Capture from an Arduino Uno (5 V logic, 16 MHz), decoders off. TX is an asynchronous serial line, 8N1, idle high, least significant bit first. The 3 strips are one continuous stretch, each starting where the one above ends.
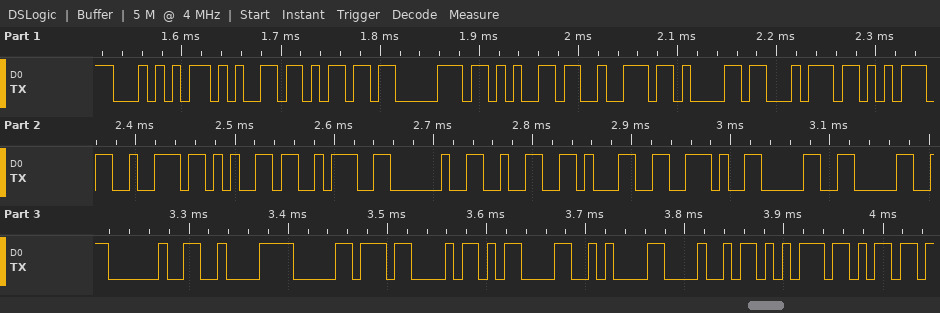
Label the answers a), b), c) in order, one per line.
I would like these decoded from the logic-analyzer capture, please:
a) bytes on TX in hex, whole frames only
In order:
a) 54 65 6D 70 65 72 61 74 75 72 65 3A 20 32 31 2E 30 30 20 C2 B0 43 0D 0A 48 75 6D
